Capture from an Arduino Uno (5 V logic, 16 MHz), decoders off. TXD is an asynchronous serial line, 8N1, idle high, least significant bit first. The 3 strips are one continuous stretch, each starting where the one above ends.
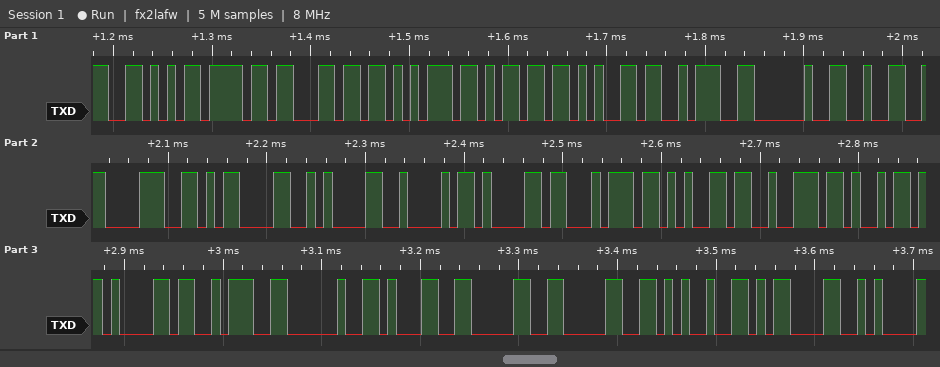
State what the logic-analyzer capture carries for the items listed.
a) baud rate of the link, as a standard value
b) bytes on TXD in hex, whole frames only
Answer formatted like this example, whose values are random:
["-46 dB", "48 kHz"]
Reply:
["115200 baud", "56 6F 6C 75 6D 65 3A 20 32 38 0D 0A 42 61 74 65 72 69 61 3A 20 31 30 30 25 0D 0A"]
